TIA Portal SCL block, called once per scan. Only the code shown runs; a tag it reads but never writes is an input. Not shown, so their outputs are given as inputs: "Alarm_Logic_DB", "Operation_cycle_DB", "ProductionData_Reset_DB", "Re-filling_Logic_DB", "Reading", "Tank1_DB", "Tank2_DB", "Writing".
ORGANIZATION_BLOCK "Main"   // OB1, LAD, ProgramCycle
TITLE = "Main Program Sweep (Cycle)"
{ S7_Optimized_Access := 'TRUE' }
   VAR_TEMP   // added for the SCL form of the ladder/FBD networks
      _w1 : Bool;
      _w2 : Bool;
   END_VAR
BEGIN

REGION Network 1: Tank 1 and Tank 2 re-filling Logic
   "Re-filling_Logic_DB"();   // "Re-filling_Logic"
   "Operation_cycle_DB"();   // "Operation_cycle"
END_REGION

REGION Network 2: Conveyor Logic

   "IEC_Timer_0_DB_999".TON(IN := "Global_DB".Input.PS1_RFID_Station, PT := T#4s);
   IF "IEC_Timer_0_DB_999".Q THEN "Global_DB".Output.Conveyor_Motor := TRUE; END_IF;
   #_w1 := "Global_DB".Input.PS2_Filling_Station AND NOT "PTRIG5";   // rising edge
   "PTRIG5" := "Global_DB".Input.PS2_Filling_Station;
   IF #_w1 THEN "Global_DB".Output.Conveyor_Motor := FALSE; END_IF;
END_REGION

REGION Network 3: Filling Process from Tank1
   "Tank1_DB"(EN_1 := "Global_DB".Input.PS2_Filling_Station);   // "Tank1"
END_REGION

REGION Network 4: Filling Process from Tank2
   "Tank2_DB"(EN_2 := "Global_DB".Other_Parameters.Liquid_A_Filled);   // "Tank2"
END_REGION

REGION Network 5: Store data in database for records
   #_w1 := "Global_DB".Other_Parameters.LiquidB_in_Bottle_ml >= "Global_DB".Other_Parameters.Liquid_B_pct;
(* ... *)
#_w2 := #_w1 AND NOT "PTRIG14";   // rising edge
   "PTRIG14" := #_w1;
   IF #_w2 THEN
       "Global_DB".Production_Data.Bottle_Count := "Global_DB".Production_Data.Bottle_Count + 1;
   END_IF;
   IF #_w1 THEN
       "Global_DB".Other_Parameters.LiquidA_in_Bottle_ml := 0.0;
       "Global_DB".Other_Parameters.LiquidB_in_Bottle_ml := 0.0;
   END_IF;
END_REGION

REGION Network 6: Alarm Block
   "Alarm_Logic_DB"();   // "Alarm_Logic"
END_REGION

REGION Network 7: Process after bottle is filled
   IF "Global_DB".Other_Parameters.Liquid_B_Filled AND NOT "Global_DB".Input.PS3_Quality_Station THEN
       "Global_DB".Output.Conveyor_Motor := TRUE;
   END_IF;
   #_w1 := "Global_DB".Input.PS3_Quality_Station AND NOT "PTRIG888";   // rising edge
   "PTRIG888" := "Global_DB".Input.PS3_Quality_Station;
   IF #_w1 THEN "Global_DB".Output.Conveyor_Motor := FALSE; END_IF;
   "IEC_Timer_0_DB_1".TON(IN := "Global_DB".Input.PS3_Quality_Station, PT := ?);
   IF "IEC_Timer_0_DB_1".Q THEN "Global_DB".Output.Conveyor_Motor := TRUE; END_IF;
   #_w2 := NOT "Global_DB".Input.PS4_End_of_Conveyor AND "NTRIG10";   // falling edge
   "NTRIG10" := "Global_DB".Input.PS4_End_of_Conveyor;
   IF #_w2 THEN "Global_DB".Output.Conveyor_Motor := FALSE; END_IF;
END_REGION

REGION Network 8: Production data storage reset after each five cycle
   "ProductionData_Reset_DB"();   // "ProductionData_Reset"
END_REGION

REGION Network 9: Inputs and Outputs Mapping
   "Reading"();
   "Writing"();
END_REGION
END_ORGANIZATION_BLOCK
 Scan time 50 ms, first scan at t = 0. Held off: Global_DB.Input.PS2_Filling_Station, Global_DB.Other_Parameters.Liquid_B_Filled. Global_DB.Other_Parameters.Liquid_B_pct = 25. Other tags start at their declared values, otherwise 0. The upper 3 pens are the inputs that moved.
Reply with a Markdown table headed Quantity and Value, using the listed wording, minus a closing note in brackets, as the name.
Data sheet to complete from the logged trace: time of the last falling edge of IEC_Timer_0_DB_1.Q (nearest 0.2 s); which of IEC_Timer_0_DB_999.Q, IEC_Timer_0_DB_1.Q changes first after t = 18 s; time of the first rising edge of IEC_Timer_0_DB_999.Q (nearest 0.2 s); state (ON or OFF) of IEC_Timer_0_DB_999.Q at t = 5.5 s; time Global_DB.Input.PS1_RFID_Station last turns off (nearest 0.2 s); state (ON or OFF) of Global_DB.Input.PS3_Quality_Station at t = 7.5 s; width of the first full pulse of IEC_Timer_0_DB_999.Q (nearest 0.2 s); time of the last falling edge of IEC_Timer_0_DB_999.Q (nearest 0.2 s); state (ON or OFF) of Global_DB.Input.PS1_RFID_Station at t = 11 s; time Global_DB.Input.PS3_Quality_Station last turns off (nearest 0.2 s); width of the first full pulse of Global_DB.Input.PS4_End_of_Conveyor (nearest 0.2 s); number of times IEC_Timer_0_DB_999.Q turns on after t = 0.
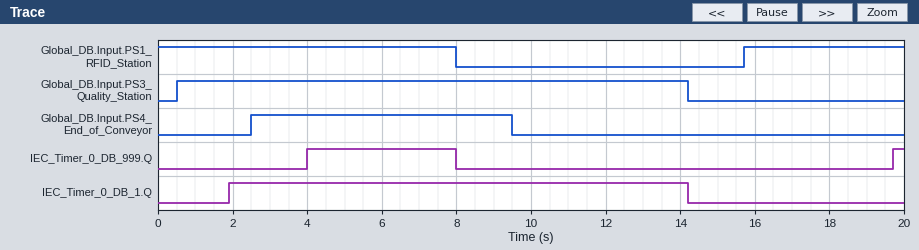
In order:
| Quantity | Value |
|---|---|
| time of the last falling edge of IEC_Timer_0_DB_1.Q | 14.2 s |
| which of IEC_Timer_0_DB_999.Q, IEC_Timer_0_DB_1.Q changes first after t = 18 s | IEC_Timer_0_DB_999.Q |
| time of the first rising edge of IEC_Timer_0_DB_999.Q | 4.0 s |
| state (ON or OFF) of IEC_Timer_0_DB_999.Q at t = 5.5 s | ON |
| time Global_DB.Input.PS1_RFID_Station last turns off | 8.0 s |
| state (ON or OFF) of Global_DB.Input.PS3_Quality_Station at t = 7.5 s | ON |
| width of the first full pulse of IEC_Timer_0_DB_999.Q | 4.0 s |
| time of the last falling edge of IEC_Timer_0_DB_999.Q | 8.0 s |
| state (ON or OFF) of Global_DB.Input.PS1_RFID_Station at t = 11 s | OFF |
| time Global_DB.Input.PS3_Quality_Station last turns off | 14.2 s |
| width of the first full pulse of Global_DB.Input.PS4_End_of_Conveyor | 7.0 s |
| number of times IEC_Timer_0_DB_999.Q turns on after t = 0 | 2 |
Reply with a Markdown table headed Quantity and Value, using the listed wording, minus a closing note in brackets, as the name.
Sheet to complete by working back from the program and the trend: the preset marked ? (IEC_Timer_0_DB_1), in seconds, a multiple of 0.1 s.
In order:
| Quantity | Value |
|---|---|
| the preset marked ? (IEC_Timer_0_DB_1), in seconds, a multiple of 0.1 s | 1.4 s |
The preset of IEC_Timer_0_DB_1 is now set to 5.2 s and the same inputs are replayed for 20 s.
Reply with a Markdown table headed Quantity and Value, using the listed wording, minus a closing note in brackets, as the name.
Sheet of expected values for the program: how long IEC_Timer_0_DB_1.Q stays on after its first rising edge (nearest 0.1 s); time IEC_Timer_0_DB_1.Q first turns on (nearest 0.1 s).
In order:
| Quantity | Value |
|---|---|
| how long IEC_Timer_0_DB_1.Q stays on after its first rising edge | 8.5 s |
| time IEC_Timer_0_DB_1.Q first turns on | 5.7 s |
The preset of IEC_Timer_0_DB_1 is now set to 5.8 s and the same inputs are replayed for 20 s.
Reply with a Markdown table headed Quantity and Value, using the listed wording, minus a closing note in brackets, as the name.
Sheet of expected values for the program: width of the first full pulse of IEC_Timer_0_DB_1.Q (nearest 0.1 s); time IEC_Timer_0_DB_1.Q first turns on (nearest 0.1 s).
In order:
| Quantity | Value |
|---|---|
| width of the first full pulse of IEC_Timer_0_DB_1.Q | 7.9 s |
| time IEC_Timer_0_DB_1.Q first turns on | 6.3 s |
